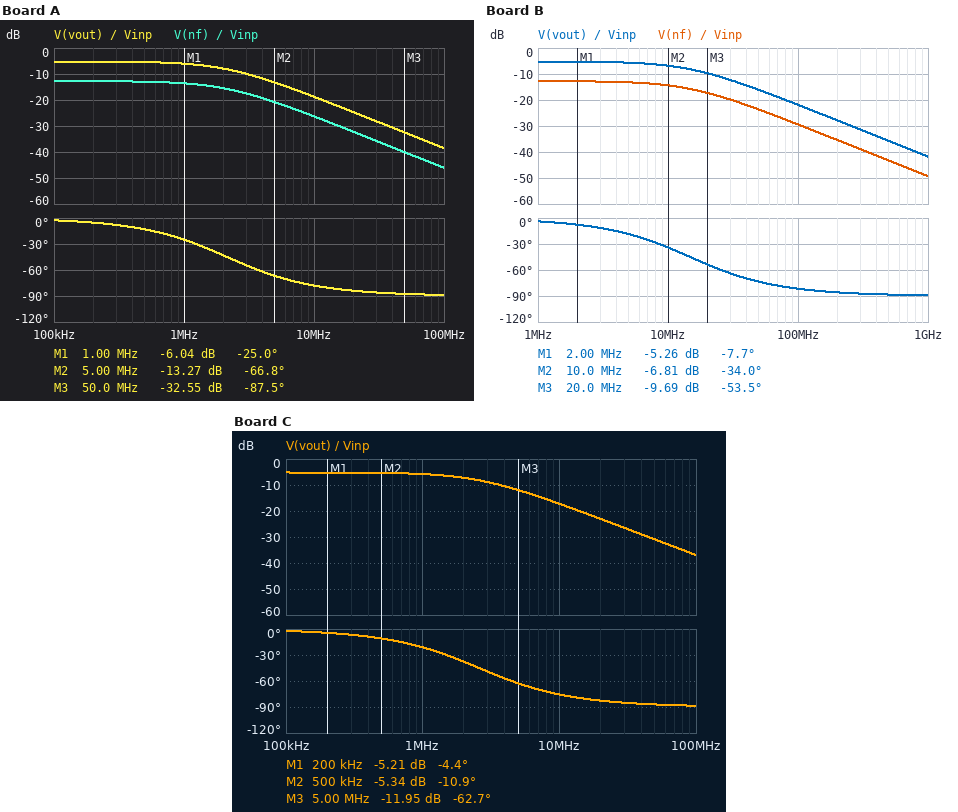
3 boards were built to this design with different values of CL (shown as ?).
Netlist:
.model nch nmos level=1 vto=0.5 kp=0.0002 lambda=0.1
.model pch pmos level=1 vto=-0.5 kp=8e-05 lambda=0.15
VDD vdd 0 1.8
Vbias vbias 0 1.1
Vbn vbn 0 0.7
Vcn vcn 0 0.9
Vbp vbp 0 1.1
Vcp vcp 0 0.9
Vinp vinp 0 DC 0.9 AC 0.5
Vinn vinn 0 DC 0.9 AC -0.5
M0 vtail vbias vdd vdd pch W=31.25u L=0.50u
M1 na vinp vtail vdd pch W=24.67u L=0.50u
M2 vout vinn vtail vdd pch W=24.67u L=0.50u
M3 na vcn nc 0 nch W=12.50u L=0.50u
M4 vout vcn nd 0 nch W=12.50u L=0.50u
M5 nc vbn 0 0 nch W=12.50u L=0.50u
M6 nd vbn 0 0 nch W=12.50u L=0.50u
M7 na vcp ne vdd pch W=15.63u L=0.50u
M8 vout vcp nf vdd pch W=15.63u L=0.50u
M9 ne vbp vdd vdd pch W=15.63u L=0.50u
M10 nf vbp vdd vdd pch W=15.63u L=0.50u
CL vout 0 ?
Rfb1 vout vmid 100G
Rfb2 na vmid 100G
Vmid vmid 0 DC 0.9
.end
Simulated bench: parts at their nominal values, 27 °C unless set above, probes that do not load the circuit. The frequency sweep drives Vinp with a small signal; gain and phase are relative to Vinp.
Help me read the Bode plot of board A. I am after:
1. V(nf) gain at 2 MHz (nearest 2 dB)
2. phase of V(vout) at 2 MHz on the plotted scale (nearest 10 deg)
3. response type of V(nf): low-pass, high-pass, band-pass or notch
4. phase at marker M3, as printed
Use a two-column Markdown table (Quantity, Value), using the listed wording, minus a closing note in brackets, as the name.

| Quantity | Value |
|---|---|
| V(nf) gain at 2 MHz | -16 dB |
| phase of V(vout) at 2 MHz on the plotted scale | -40 deg |
| response type of V(nf): low-pass, high-pass, band-pass or notch | low-pass |
| phase at marker M3, as printed | -87.5 deg |
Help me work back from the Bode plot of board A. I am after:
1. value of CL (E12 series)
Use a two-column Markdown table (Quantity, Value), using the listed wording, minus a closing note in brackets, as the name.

| Quantity | Value |
|---|---|
| value of CL | 4.7 pF |
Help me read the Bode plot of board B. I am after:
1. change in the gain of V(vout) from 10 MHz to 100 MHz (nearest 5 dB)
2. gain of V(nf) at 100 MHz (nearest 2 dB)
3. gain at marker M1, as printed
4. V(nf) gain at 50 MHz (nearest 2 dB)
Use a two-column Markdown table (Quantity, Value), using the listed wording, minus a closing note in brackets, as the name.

| Quantity | Value |
|---|---|
| change in the gain of V(vout) from 10 MHz to 100 MHz | -15 dB |
| gain of V(nf) at 100 MHz | -30 dB |
| gain at marker M1, as printed | -5.26 dB |
| V(nf) gain at 50 MHz | -24 dB |
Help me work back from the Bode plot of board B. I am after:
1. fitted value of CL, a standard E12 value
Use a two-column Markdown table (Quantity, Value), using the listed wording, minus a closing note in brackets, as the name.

| Quantity | Value |
|---|---|
| fitted value of CL, a standard E12 value | 680 fF |
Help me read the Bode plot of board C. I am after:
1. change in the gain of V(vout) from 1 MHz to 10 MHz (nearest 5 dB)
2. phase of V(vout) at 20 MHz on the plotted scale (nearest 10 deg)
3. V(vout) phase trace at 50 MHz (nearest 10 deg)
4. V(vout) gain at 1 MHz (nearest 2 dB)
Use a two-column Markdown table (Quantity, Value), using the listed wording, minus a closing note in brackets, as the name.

| Quantity | Value |
|---|---|
| change in the gain of V(vout) from 1 MHz to 10 MHz | -10 dB |
| phase of V(vout) at 20 MHz on the plotted scale | -80 deg |
| V(vout) phase trace at 50 MHz | -90 deg |
| V(vout) gain at 1 MHz | -6 dB |
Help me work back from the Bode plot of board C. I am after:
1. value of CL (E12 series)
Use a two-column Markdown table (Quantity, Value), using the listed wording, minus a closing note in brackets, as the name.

| Quantity | Value |
|---|---|
| value of CL | 3.9 pF |
